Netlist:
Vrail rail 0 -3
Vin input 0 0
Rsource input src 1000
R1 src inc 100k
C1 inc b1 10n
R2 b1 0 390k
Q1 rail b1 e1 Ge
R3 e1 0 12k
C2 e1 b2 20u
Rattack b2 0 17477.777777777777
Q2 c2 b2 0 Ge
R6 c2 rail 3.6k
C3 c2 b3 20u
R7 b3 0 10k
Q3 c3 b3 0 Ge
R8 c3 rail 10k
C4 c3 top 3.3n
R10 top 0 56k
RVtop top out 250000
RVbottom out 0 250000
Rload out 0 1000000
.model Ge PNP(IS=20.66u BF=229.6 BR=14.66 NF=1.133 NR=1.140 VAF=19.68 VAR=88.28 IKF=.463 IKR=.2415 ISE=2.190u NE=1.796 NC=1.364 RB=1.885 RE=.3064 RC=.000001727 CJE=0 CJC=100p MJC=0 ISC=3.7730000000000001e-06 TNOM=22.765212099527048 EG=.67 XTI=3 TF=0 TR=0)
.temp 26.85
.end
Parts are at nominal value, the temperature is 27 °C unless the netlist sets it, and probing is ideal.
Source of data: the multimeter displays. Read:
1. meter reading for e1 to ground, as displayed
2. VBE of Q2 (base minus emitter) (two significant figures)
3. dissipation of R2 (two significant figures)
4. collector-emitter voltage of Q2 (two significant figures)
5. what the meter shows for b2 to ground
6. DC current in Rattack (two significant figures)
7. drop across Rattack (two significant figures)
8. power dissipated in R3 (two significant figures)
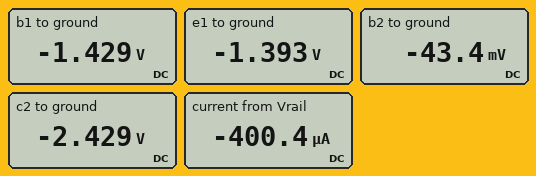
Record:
-1.393 V
-43 mV
5.2 µW
-2.4 V
-43.4 mV
2.5 µA
43 mV
160 µW
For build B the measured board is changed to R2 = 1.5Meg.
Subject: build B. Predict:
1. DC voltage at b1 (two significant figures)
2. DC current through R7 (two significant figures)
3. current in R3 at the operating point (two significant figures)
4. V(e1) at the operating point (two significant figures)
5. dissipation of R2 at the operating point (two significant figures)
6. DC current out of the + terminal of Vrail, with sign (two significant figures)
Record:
-2.2 V
3.6 µA
180 µA
-2.1 V
3.1 µW
-460 µA
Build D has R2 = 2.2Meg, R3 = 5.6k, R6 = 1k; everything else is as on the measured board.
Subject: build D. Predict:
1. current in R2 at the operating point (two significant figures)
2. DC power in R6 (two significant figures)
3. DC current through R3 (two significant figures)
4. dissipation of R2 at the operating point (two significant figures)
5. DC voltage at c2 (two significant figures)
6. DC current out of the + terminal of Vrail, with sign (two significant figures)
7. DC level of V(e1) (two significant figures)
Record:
570 nA
26 µW
210 µA
710 nW
-2.8 V
-500 µA
-1.2 V
